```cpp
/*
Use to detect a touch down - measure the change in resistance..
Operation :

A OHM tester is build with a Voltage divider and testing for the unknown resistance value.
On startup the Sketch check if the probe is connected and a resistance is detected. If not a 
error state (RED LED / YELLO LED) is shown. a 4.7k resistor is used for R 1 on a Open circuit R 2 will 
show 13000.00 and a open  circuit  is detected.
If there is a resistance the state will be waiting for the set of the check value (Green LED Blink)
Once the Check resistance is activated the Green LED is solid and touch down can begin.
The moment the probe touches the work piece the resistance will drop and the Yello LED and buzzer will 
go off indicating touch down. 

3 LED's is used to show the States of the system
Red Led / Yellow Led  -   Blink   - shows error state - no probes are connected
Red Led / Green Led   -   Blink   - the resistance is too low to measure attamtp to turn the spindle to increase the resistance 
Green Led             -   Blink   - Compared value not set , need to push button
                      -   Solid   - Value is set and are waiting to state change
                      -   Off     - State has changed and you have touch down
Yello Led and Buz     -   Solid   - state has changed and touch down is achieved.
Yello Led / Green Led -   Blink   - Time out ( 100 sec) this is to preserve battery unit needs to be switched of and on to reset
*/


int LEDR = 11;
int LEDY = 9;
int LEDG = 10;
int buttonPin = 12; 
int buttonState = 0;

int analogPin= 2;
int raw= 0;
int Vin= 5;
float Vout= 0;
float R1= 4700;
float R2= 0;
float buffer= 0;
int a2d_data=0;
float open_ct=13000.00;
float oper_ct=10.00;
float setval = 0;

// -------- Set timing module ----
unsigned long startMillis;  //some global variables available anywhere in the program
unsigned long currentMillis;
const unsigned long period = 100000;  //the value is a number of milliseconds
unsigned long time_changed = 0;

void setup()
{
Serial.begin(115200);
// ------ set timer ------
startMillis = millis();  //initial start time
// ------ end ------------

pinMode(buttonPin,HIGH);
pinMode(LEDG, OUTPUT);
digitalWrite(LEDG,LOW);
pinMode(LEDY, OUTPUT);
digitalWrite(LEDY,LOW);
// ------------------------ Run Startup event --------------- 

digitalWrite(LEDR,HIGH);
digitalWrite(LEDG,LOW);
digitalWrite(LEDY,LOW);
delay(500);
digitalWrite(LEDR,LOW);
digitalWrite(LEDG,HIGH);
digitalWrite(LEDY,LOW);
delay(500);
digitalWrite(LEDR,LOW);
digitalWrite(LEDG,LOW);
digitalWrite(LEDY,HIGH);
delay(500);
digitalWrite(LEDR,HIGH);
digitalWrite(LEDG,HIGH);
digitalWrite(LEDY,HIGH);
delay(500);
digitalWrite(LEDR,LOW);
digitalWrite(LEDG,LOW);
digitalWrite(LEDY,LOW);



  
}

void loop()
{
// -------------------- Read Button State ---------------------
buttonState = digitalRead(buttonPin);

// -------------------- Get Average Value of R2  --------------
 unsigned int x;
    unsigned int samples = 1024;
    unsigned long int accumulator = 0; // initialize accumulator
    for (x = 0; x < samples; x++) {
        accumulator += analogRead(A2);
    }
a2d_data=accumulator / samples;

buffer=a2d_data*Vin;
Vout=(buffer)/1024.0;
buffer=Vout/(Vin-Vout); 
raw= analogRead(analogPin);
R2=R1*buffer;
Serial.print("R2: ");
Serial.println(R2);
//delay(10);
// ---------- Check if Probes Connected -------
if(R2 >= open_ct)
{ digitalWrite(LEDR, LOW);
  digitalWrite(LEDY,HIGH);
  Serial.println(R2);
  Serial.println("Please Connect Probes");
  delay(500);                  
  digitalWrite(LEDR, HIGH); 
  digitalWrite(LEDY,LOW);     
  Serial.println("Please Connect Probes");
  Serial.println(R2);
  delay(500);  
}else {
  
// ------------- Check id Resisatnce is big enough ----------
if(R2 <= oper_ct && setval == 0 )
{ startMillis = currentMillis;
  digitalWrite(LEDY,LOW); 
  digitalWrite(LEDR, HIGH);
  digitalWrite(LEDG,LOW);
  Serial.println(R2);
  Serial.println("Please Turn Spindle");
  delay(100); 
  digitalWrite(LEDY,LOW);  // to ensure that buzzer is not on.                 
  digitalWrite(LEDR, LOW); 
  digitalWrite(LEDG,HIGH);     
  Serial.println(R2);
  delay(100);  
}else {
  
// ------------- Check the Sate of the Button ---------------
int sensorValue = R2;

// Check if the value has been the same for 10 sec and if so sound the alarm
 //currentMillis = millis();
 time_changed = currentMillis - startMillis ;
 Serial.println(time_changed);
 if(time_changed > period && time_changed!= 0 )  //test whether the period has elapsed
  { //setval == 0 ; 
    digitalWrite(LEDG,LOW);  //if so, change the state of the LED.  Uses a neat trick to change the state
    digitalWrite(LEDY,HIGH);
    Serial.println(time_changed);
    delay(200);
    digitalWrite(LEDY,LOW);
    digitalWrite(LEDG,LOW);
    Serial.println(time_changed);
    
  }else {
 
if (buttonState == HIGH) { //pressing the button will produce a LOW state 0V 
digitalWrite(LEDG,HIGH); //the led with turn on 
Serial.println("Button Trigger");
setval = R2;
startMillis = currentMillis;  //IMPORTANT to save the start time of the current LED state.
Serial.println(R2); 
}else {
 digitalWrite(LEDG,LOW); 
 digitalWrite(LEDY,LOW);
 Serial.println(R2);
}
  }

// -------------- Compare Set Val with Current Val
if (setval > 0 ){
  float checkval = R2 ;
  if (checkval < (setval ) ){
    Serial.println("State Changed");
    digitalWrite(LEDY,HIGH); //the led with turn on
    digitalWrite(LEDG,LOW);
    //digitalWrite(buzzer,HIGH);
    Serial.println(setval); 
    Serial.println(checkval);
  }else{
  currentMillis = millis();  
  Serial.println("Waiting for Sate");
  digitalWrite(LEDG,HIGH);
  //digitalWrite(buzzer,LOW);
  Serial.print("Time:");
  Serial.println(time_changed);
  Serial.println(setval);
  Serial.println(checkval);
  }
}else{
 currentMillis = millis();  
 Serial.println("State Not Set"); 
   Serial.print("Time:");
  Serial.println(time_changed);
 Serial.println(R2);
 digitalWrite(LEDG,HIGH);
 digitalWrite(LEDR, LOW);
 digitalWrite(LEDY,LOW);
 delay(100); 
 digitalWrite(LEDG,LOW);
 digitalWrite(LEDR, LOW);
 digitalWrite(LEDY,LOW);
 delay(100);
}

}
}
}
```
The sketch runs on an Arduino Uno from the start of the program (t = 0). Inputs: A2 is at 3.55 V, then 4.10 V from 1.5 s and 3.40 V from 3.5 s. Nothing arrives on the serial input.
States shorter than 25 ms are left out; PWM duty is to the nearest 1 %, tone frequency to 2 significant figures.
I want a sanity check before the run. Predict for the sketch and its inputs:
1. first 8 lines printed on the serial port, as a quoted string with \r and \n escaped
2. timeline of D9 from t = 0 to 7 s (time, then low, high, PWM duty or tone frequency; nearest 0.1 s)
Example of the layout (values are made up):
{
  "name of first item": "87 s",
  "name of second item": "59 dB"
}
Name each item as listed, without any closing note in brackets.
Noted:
{
  "first 8 lines printed on the serial port, as a quoted string with \\r and \\n escaped": "\"R2: 21315.14\\r\\n21315.14\\r\\nPlease Connect Probes\\r\\nPlease Connect Probes\\r\\n21315.14\\r\\nR2: 21315.14\\r\\n21315.14\\r\\nPlease Connect Probes\\r\\n\"",
  "timeline of D9 from t = 0 to 7 s": "0 s low; 1 s high; 2 s low; 2.1 s high; 2.6 s low; 3.2 s high; 3.7 s low"
}
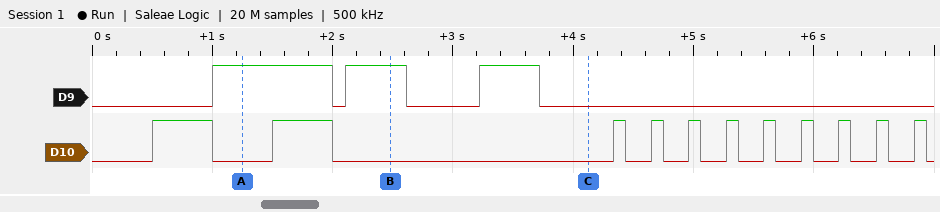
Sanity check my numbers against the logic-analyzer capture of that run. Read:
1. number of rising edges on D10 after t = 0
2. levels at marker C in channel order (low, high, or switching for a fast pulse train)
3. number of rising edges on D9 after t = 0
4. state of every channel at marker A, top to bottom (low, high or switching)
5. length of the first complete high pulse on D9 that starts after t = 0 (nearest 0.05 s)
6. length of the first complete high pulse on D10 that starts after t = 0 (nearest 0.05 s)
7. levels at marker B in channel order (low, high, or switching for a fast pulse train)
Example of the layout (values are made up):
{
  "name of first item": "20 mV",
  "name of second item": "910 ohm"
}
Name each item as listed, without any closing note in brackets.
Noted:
{
  "number of rising edges on D10 after t = 0": "11",
  "levels at marker C in channel order": "D9 low, D10 low",
  "number of rising edges on D9 after t = 0": "3",
  "state of every channel at marker A, top to bottom": "D9 high, D10 low",
  "length of the first complete high pulse on D9 that starts after t = 0": "1.00 s",
  "length of the first complete high pulse on D10 that starts after t = 0": "0.50 s",
  "levels at marker B in channel order": "D9 high, D10 low"
}
